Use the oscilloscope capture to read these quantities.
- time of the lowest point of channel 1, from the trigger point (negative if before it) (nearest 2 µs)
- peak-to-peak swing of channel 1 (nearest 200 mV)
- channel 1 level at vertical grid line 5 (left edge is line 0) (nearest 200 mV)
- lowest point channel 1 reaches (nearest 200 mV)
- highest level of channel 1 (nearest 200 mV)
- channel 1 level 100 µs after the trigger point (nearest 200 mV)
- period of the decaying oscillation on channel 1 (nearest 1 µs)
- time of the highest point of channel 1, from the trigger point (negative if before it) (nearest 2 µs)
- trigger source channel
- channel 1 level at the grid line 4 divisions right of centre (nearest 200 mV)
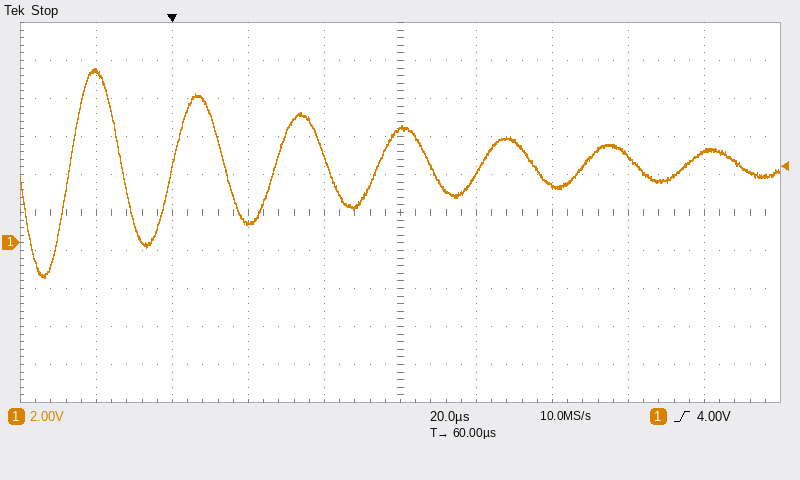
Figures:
-34 µs
11.0 V
6.0 V
-1.8 V
9.2 V
3.0 V
27 µs
-20 µs
channel 1
4.8 V
